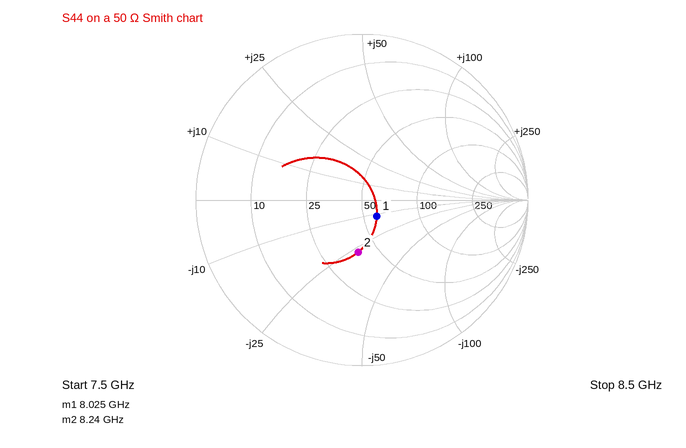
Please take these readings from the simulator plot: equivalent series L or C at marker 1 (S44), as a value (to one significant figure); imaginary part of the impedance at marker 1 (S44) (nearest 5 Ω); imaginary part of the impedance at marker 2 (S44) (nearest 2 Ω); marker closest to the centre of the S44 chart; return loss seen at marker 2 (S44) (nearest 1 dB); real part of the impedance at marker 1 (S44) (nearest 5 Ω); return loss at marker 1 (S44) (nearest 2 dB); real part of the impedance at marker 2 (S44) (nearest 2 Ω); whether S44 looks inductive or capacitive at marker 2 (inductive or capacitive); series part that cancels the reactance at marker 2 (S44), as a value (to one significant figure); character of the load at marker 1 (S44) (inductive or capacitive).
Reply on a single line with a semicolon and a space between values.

2 pF; -10 Ω; -28 Ω; marker 1; 10 dB; 60 Ω; 18 dB; 40 Ω; capacitive; 500 pH; capacitive
